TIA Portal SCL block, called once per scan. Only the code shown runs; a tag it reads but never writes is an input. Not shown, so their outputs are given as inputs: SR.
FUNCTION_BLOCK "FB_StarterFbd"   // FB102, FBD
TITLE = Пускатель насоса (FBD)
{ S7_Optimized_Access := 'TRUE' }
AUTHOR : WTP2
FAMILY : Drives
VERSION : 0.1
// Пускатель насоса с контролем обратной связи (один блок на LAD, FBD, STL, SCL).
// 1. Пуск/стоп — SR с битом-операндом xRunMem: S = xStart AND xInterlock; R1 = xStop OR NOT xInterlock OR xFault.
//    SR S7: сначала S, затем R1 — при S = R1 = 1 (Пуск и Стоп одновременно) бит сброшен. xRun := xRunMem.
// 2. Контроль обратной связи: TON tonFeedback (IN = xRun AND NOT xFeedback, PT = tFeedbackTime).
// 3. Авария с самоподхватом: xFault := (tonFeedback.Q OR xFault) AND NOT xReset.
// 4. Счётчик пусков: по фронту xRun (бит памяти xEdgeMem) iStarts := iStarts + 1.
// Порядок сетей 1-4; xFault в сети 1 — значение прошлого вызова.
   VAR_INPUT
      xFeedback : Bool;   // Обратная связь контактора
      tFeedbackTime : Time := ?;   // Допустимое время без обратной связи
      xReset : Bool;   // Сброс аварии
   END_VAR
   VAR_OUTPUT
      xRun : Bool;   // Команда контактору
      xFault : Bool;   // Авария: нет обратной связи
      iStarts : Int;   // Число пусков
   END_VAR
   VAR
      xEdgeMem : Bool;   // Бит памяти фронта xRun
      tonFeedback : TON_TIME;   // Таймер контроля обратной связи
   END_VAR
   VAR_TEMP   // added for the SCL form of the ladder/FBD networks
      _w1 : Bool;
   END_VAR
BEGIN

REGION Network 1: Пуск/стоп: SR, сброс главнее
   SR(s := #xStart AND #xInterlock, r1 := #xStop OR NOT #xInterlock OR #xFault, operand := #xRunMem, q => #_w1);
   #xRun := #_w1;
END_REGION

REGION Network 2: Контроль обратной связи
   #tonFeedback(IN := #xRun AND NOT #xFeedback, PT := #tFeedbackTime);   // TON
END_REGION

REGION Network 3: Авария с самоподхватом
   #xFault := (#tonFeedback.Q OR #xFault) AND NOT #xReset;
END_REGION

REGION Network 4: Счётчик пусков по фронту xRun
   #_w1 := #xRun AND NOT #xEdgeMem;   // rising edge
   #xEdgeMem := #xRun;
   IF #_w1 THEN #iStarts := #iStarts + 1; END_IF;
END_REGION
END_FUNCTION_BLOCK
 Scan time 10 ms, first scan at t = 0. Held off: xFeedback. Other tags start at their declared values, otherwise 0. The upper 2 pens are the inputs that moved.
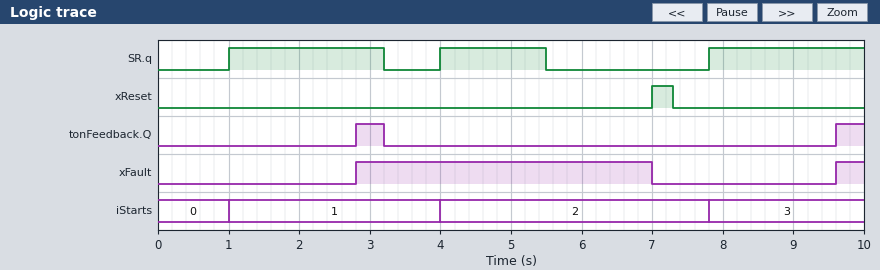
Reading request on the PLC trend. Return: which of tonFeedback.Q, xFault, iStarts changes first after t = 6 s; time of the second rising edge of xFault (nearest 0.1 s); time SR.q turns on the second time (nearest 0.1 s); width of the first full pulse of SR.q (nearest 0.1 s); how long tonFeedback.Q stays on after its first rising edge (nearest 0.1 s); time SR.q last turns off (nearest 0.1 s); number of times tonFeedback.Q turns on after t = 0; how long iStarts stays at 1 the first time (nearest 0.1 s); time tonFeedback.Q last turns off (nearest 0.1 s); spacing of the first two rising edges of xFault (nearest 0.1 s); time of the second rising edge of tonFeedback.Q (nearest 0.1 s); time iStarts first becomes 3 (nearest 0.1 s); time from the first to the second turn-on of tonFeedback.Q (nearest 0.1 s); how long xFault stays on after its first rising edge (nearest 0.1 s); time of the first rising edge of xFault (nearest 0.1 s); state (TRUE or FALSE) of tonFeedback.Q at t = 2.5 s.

xFault
9.6 s
4.0 s
2.2 s
0.4 s
5.5 s
2
3.0 s
3.2 s
6.8 s
9.6 s
7.8 s
6.8 s
4.2 s
2.8 s
FALSE
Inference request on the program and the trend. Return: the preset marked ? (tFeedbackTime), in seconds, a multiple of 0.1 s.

1.8 s
